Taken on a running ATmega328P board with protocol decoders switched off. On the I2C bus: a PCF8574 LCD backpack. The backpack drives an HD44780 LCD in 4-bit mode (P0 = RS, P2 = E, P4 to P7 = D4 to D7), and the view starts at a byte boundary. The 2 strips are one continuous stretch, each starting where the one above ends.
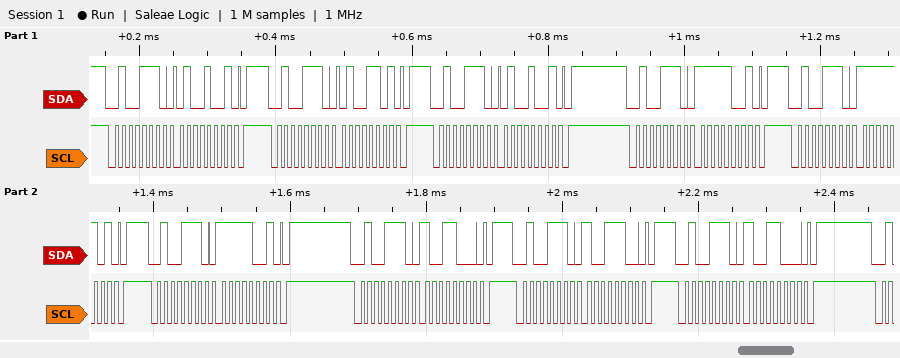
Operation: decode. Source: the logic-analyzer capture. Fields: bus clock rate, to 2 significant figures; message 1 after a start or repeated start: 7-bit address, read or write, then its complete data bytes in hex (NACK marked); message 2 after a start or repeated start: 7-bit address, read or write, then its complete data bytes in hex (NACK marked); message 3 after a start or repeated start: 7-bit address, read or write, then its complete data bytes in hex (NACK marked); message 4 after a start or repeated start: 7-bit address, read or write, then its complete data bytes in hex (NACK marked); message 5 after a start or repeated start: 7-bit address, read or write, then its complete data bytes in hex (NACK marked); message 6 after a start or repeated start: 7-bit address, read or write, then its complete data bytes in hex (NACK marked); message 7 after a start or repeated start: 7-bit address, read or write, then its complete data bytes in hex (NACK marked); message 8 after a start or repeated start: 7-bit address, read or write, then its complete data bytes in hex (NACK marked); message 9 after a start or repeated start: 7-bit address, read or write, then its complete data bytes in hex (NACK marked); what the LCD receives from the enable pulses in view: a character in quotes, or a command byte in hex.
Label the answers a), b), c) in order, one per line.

a) 100 kHz
b) 0x27 write: 49
c) 0x27 write: 4D
d) 0x27 write: 49
e) 0x27 write: F9
f) 0x27 write: FD
g) 0x27 write: F9
h) 0x27 write: 98
i) 0x27 write: 9C
j) 0x27 write: 98
k) 'O'
